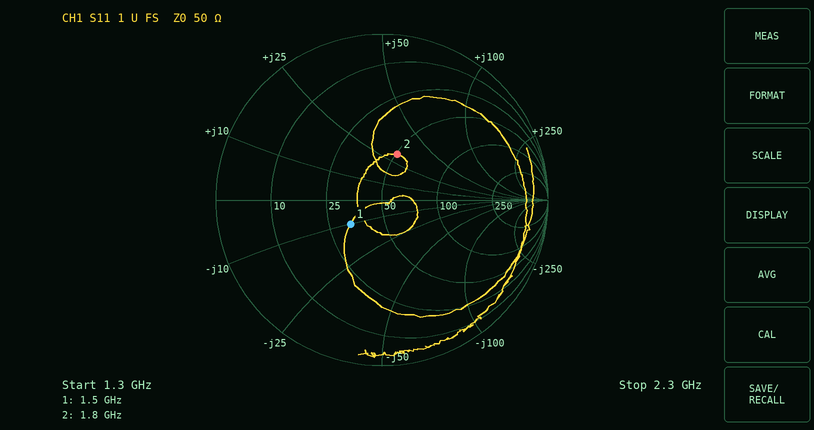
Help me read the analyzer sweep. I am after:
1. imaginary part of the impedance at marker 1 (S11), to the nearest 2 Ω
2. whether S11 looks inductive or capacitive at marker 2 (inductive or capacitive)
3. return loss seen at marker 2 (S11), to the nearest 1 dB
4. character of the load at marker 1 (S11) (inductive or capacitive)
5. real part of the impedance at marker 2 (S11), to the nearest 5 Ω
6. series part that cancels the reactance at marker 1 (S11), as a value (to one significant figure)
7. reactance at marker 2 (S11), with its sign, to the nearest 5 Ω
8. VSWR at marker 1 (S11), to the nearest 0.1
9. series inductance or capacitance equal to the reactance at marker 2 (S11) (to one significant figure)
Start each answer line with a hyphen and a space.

- -10 Ω
- inductive
- 11 dB
- capacitive
- 50 Ω
- 1 nH
- +30 Ω
- 1.6
- 3 nH
